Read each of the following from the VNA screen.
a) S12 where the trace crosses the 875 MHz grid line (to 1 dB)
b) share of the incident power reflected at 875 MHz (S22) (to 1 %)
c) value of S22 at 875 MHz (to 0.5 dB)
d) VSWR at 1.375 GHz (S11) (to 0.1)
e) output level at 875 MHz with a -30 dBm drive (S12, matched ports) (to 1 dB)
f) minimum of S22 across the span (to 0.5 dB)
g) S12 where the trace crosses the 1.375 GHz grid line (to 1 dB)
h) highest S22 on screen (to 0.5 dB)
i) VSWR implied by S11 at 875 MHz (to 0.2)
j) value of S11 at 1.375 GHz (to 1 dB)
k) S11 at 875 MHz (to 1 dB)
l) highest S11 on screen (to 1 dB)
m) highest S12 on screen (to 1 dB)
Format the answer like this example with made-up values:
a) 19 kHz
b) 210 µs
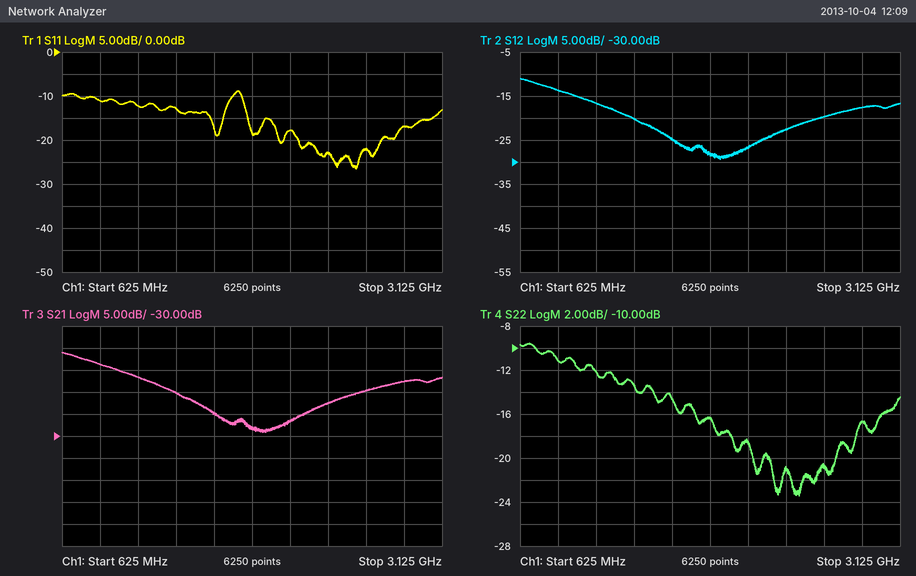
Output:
a) -14 dB
b) 8 %
c) -11.0 dB
d) 1.6
e) -44 dBm
f) -23.5 dB
g) -20 dB
h) -9.5 dB
i) 1.8
j) -13 dB
k) -11 dB
l) -9 dB
m) -11 dB
